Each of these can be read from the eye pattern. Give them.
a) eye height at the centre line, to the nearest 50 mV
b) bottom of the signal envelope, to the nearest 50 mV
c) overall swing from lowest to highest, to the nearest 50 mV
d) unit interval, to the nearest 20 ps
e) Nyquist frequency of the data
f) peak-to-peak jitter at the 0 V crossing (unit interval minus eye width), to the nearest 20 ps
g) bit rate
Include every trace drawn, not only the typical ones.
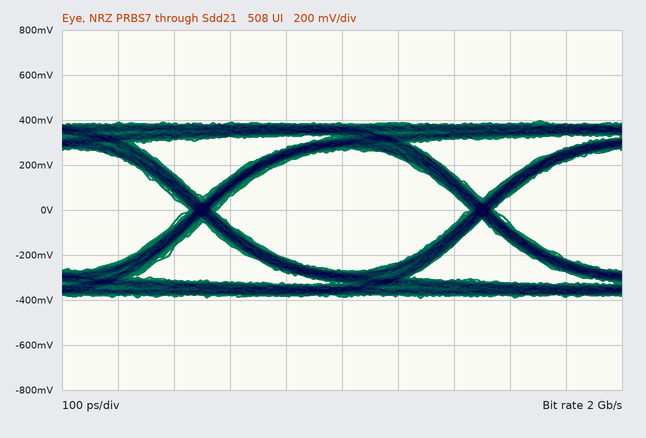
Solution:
550 mV
-400 mV
800 mV
500 ps
1 GHz
40 ps
2 Gb/s
